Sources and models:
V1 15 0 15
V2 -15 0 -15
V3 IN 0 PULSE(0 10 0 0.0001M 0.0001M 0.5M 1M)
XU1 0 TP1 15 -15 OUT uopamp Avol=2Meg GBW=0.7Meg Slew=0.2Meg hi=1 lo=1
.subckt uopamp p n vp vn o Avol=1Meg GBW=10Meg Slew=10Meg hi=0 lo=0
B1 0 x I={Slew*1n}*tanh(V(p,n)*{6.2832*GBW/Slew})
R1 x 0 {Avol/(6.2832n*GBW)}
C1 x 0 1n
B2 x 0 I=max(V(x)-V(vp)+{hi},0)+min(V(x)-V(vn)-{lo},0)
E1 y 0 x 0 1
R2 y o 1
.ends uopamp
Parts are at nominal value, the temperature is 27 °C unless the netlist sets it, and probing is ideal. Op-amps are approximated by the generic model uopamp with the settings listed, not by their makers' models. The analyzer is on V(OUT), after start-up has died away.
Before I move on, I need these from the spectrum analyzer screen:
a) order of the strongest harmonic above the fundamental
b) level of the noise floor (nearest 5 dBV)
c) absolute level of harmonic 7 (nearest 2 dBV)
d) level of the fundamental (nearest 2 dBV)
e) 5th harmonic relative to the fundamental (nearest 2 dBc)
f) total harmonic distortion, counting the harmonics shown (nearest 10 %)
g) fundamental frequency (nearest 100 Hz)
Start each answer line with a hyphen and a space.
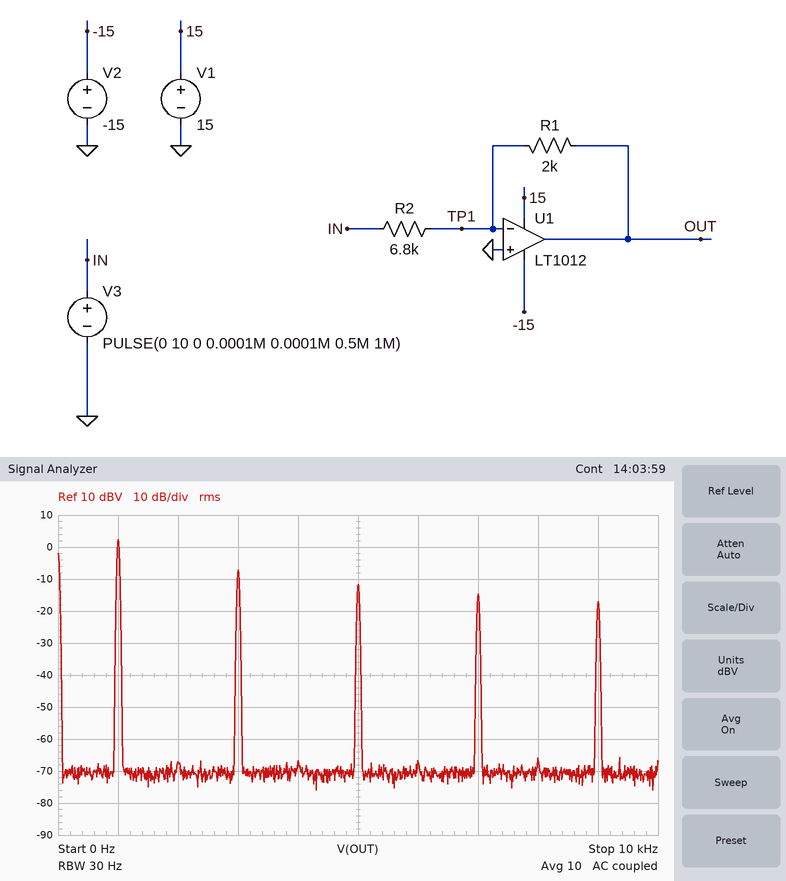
- 3
- -70 dBV
- -14 dBV
- 2 dBV
- -14 dBc
- 40 %
- 1.0 kHz
